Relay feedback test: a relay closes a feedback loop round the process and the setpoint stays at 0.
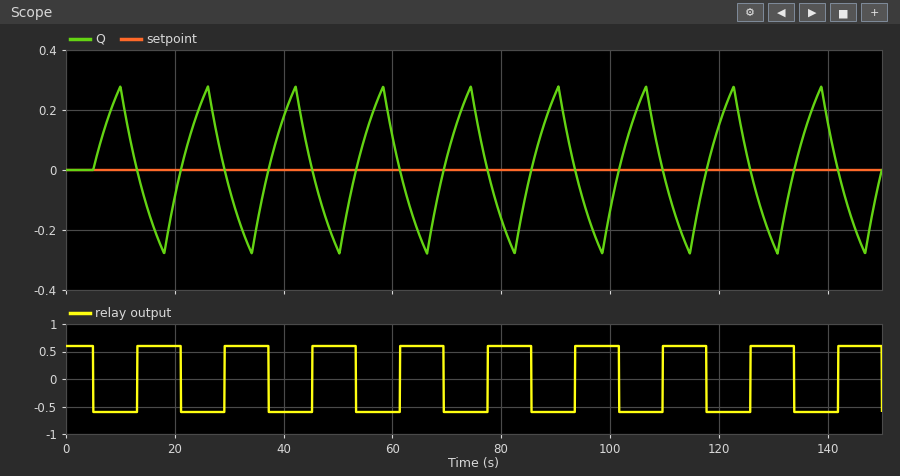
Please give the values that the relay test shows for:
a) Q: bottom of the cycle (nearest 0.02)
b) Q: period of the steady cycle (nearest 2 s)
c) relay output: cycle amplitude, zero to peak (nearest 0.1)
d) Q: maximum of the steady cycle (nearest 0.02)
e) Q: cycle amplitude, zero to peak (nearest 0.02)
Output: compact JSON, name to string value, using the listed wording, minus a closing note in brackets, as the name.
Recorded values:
{"Q: bottom of the cycle": "-0.28", "Q: period of the steady cycle": "16 s", "relay output: cycle amplitude, zero to peak": "0.6", "Q: maximum of the steady cycle": "0.28", "Q: cycle amplitude, zero to peak": "0.28"}
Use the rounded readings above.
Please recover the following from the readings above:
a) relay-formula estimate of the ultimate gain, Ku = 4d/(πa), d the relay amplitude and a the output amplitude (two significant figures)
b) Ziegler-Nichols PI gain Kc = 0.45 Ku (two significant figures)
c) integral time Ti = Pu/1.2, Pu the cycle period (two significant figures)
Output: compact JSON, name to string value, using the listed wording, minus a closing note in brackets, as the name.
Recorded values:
{"relay-formula estimate of the ultimate gain, Ku = 4d/(πa), d the relay amplitude and a the output amplitude": "2.7", "Ziegler-Nichols PI gain Kc = 0.45 Ku": "1.2", "integral time Ti = Pu/1.2, Pu the cycle period": "13 s"}
